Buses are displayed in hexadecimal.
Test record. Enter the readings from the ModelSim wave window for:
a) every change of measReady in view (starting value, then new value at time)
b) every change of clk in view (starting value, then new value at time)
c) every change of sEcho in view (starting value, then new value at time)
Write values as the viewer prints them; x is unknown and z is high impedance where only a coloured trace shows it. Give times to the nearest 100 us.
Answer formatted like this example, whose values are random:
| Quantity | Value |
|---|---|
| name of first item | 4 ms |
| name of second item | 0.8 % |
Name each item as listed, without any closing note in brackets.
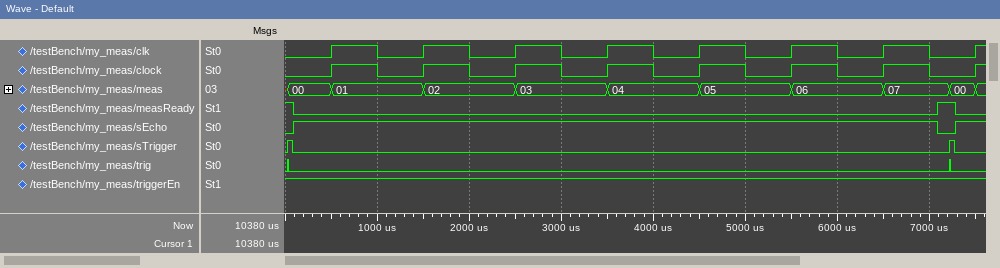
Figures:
| Quantity | Value |
|---|---|
| every change of measReady in view | 1, 0 at 100 us, 1 at 7100 us, 0 at 7300 us |
| every change of clk in view | 0, 1 at 500 us, 0 at 1000 us, 1 at 1500 us, 0 at 2000 us, 1 at 2500 us, 0 at 3000 us, 1 at 3500 us, 0 at 4000 us, 1 at 4500 us, 0 at 5000 us, 1 at 5500 us, 0 at 6000 us, 1 at 6500 us, 0 at 7000 us, 1 at 7500 us |
| every change of sEcho in view | 0, 1 at 100 us, 0 at 7100 us, 1 at 7300 us |
